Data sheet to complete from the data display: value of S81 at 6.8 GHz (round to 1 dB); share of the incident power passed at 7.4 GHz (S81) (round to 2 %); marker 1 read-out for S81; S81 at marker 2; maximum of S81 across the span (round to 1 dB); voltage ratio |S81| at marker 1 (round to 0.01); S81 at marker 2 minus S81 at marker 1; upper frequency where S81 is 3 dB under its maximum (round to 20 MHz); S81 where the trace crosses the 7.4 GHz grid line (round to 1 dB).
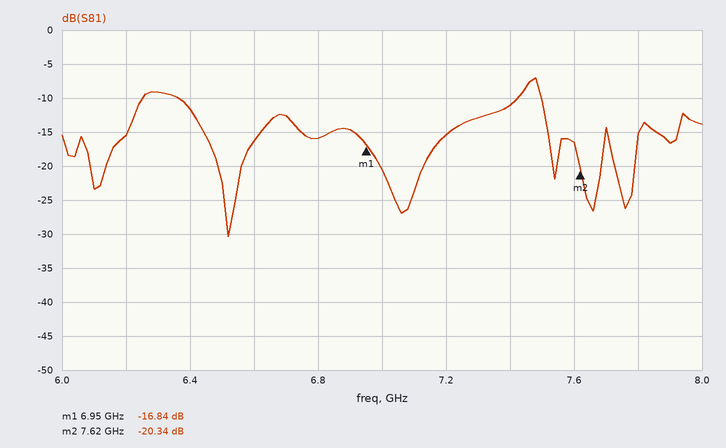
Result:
-16 dB
8 %
-16.84 dB
-20.34 dB
-7 dB
0.14
-3.50 dB
7.50 GHz
-11 dB
